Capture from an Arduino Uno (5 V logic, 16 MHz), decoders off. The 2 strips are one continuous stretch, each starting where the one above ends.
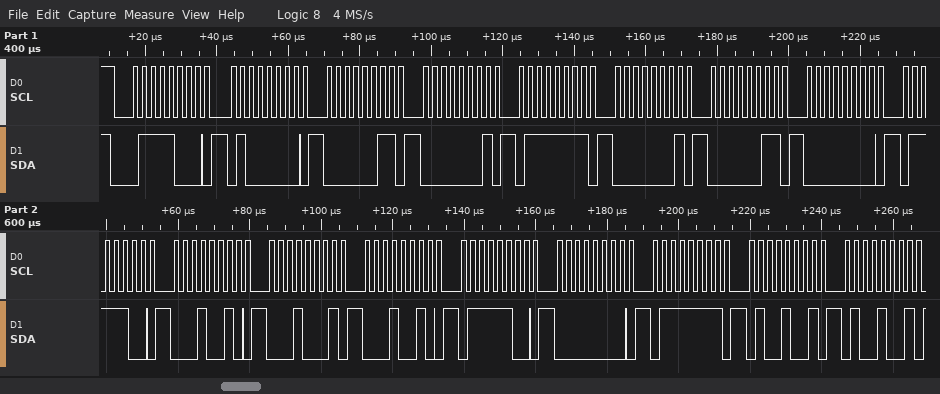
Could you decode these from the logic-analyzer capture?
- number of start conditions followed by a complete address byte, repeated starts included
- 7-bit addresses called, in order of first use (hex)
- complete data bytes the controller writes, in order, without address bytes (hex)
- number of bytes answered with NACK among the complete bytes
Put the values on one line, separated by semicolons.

1; 0x3C; 40 03 01 7F 01 03 00 7C 12 11 12 7C 00 7F 49 49; 0
